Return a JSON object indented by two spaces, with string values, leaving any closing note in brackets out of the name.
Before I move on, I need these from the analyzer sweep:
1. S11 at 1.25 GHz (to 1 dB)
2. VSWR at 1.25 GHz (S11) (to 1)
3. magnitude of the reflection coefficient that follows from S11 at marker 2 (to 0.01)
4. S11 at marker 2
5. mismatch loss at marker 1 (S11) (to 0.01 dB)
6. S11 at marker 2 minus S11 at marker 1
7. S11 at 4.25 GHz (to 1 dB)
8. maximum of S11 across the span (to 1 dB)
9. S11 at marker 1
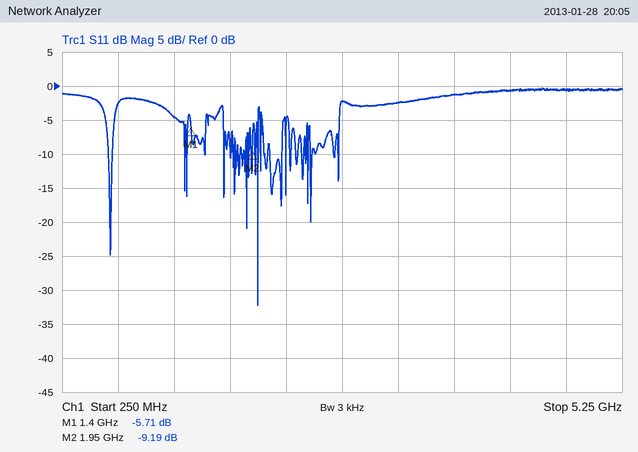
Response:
{
  "S11 at 1.25 GHz": "-5 dB",
  "VSWR at 1.25 GHz (S11)": "4",
  "magnitude of the reflection coefficient that follows from S11 at marker 2": "0.35",
  "S11 at marker 2": "-9.19 dB",
  "mismatch loss at marker 1 (S11)": "1.36 dB",
  "S11 at marker 2 minus S11 at marker 1": "-3.48 dB",
  "S11 at 4.25 GHz": "-1 dB",
  "maximum of S11 across the span": "0 dB",
  "S11 at marker 1": "-5.71 dB"
}
